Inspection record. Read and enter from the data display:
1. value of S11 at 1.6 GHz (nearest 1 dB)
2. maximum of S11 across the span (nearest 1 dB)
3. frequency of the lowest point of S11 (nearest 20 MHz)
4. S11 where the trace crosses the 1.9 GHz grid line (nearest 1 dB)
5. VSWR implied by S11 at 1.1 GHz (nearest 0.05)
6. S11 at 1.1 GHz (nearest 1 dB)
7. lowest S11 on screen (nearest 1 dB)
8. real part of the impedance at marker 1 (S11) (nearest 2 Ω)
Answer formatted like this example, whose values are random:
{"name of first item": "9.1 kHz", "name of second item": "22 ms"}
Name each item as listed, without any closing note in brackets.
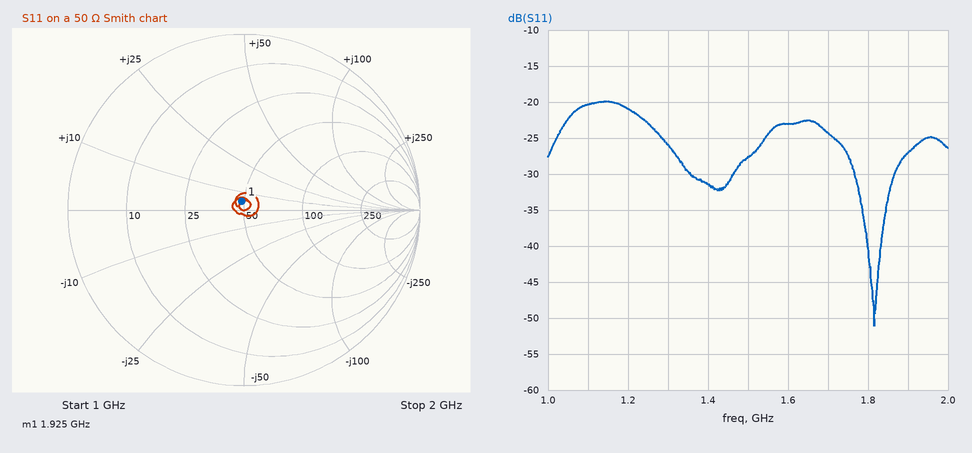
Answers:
{"value of S11 at 1.6 GHz": "-23 dB", "maximum of S11 across the span": "-20 dB", "frequency of the lowest point of S11": "1.82 GHz", "S11 where the trace crosses the 1.9 GHz grid line": "-27 dB", "VSWR implied by S11 at 1.1 GHz": "1.20", "S11 at 1.1 GHz": "-20 dB", "lowest S11 on screen": "-51 dB", "real part of the impedance at marker 1 (S11)": "48 Ω"}
